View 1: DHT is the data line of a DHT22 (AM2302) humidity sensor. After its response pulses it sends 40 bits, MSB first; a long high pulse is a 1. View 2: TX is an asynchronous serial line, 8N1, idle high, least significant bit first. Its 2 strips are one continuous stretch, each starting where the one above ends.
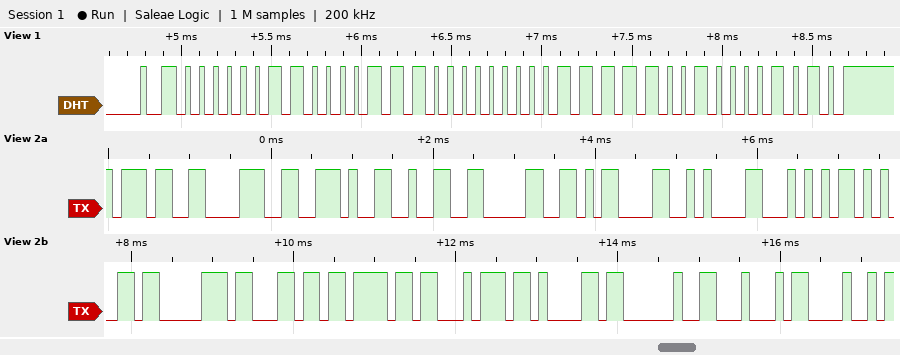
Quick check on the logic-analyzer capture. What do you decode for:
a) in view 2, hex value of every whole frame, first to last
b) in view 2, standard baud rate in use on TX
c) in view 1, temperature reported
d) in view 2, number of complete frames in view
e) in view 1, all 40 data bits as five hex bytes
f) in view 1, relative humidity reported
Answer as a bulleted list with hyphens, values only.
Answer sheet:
- 37 38 2E 32 30 0D 0A 54 65 70 6C 6F 74 61 20 44 48
- 9600 baud
- 24.9 °C
- 17
- 03 0E 00 F9 0A
- 78.2 %
